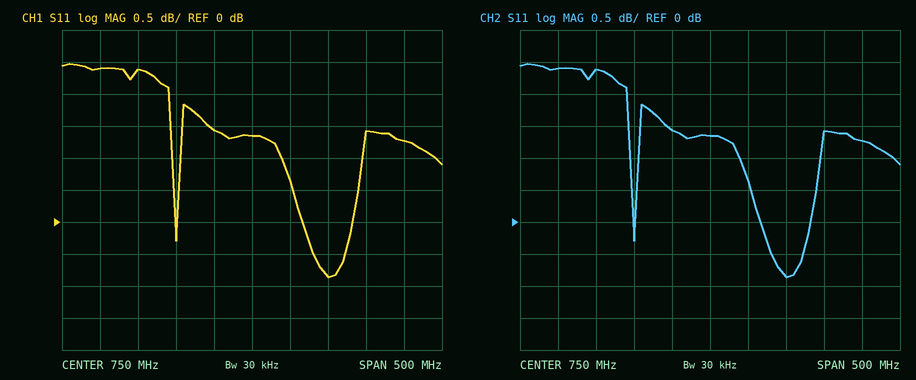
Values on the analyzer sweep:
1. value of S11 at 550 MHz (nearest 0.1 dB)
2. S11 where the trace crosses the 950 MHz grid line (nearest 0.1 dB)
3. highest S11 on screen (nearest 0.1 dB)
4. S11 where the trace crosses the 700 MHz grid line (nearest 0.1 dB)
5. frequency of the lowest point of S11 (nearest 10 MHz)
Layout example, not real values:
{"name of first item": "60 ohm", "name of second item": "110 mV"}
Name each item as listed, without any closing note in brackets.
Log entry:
{"value of S11 at 550 MHz": "2.4 dB", "S11 where the trace crosses the 950 MHz grid line": "1.3 dB", "highest S11 on screen": "2.5 dB", "S11 where the trace crosses the 700 MHz grid line": "1.4 dB", "frequency of the lowest point of S11": "850 MHz"}
